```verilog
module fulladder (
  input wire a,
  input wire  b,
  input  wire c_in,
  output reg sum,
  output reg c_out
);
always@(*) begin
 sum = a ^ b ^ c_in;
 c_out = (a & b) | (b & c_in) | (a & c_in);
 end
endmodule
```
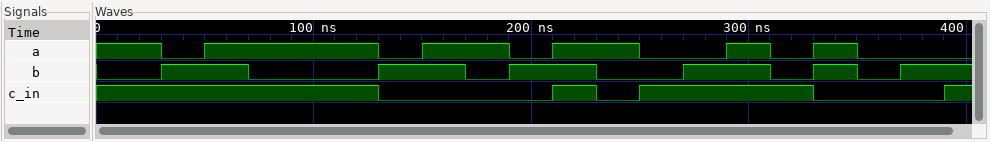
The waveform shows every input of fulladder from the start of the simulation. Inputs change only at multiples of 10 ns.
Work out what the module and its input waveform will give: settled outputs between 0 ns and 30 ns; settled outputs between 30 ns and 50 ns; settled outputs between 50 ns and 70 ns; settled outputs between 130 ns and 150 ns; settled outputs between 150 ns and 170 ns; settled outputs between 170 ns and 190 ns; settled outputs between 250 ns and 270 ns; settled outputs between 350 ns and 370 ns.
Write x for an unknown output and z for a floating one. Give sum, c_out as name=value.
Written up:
sum=0, c_out=1
sum=0, c_out=1
sum=1, c_out=1
sum=1, c_out=0
sum=0, c_out=1
sum=1, c_out=0
sum=1, c_out=0
sum=0, c_out=0
